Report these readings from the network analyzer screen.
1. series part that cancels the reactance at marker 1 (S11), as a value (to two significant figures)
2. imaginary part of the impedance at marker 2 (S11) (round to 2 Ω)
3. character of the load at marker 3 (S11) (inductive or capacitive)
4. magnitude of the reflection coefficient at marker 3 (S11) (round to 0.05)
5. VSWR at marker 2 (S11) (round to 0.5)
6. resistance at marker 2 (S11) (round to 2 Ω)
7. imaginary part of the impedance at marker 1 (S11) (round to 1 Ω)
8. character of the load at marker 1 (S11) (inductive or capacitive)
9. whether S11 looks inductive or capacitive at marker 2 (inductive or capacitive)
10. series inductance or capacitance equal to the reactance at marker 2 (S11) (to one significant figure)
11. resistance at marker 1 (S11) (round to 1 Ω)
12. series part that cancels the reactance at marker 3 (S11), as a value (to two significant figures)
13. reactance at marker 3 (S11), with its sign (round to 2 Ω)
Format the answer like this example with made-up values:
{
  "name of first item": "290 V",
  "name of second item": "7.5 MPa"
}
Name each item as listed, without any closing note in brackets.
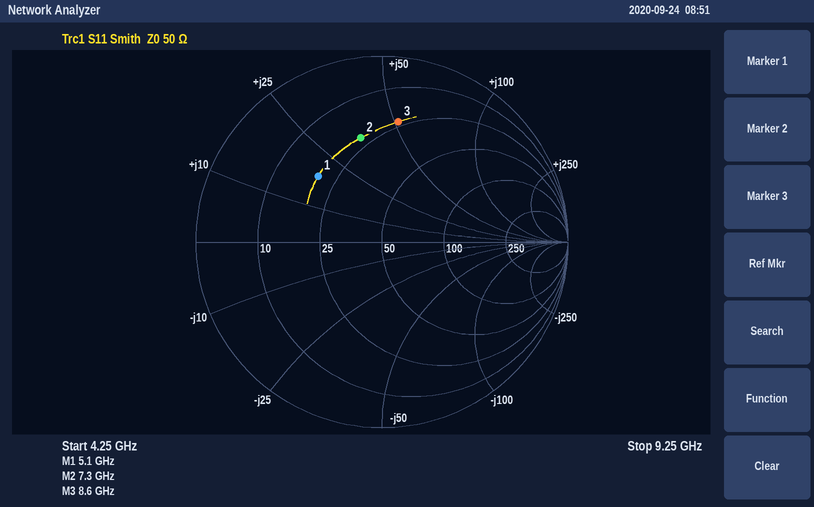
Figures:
{
  "series part that cancels the reactance at marker 1 (S11), as a value": "1.7 pF",
  "imaginary part of the impedance at marker 2 (S11)": "+36 Ω",
  "character of the load at marker 3 (S11)": "inductive",
  "magnitude of the reflection coefficient at marker 3 (S11)": "0.65",
  "VSWR at marker 2 (S11)": "3.5",
  "resistance at marker 2 (S11)": "22 Ω",
  "imaginary part of the impedance at marker 1 (S11)": "+18 Ω",
  "character of the load at marker 1 (S11)": "inductive",
  "whether S11 looks inductive or capacitive at marker 2": "inductive",
  "series inductance or capacitance equal to the reactance at marker 2 (S11)": "800 pH",
  "resistance at marker 1 (S11)": "20 Ω",
  "series part that cancels the reactance at marker 3 (S11), as a value": "360 fF",
  "reactance at marker 3 (S11), with its sign": "+52 Ω"
}
